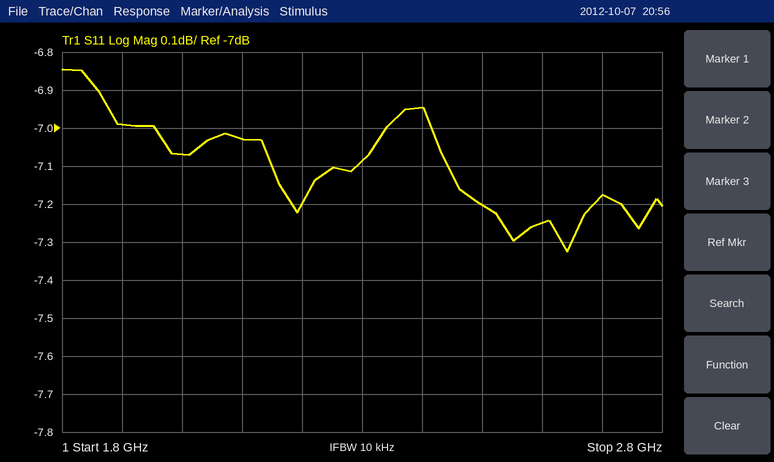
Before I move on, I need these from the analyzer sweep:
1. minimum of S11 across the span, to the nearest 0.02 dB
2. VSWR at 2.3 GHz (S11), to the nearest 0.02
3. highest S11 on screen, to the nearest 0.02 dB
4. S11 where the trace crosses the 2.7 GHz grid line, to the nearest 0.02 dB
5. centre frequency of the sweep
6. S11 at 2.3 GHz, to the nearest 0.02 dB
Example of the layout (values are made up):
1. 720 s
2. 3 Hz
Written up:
1. -7.32 dB
2. 2.58
3. -6.84 dB
4. -7.18 dB
5. 2.3 GHz
6. -7.08 dB
